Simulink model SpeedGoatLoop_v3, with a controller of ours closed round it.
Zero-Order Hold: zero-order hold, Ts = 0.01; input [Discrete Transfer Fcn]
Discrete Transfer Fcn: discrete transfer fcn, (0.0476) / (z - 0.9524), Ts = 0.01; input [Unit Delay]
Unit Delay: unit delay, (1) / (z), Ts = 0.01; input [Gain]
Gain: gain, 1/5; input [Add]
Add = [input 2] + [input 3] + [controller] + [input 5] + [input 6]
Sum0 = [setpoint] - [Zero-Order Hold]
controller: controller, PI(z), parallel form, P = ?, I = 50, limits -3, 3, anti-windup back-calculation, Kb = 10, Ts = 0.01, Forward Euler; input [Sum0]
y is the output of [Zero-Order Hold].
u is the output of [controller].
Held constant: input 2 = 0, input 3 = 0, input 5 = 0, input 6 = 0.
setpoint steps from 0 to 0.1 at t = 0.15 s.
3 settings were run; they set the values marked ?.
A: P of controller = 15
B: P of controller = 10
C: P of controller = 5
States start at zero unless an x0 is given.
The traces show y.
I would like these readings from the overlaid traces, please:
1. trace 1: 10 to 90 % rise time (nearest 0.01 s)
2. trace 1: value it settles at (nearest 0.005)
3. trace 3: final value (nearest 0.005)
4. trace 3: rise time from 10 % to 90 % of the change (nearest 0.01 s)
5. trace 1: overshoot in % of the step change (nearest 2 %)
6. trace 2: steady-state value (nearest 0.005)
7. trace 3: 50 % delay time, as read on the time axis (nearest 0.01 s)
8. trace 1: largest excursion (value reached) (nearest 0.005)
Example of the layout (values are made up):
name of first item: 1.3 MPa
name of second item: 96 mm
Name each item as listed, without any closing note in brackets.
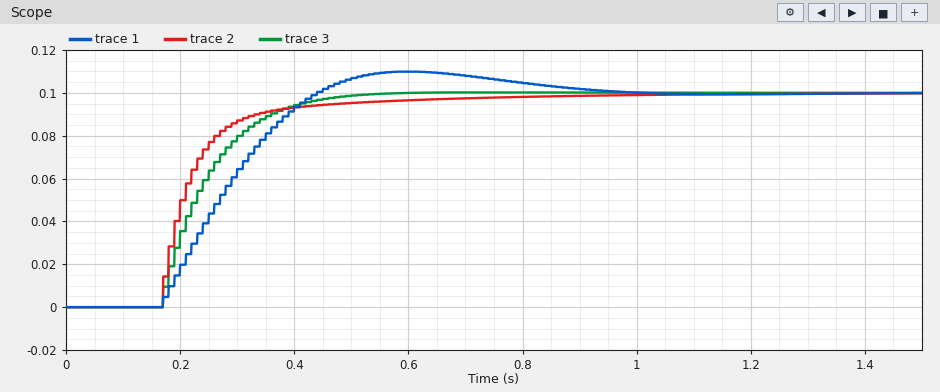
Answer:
trace 1: 10 to 90 % rise time: 0.20 s
trace 1: value it settles at: 0.100
trace 3: final value: 0.100
trace 3: rise time from 10 % to 90 % of the change: 0.18 s
trace 1: overshoot in % of the step change: 10 %
trace 2: steady-state value: 0.100
trace 3: 50 % delay time, as read on the time axis: 0.23 s
trace 1: largest excursion (value reached): 0.110
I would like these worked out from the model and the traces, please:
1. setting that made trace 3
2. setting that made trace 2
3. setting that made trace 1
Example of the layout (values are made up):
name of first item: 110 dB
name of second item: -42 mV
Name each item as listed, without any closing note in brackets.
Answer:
setting that made trace 3: B
setting that made trace 2: A
setting that made trace 1: C
